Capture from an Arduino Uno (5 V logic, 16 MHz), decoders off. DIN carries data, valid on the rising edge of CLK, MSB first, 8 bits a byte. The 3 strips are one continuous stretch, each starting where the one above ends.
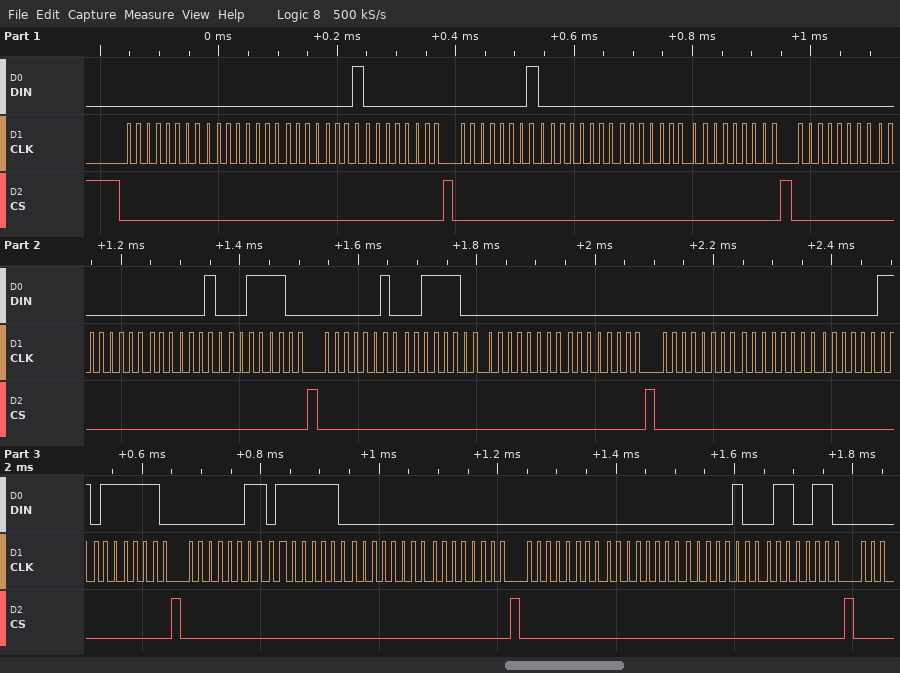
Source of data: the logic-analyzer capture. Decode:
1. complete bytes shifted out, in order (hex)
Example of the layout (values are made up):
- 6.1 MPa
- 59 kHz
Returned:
- 0x00 0x00 0x01 0x00 0x01 0x00 0x00 0x00 0x00 0x00 0x02 0x3C 0x02 0x3C 0x00 0x00 0x00 0x00 0x03 0x7E 0x03 0x7E 0x00 0x00 0x00 0x00 0x04 0x66
